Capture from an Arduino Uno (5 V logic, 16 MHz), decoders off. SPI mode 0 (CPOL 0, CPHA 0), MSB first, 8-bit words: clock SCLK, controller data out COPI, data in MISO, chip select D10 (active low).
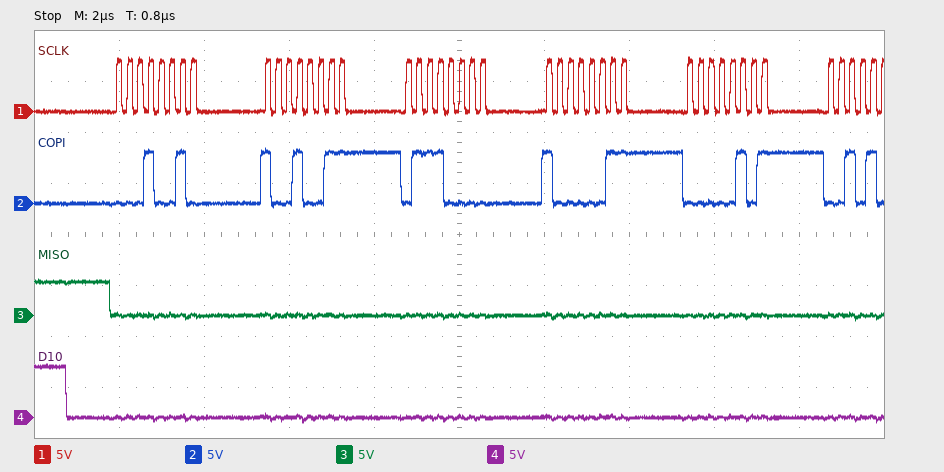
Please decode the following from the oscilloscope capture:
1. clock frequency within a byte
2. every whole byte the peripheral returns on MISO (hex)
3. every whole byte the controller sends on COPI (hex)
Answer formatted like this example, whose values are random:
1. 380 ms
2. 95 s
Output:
1. 4 MHz
2. 0x00 0x00 0x00 0x00 0x00
3. 0x12 0x93 0x70 0x83 0x05
